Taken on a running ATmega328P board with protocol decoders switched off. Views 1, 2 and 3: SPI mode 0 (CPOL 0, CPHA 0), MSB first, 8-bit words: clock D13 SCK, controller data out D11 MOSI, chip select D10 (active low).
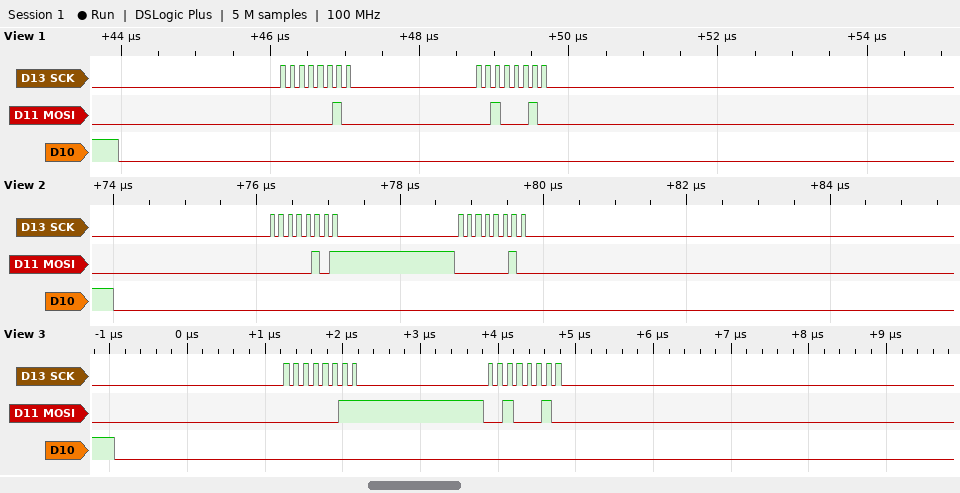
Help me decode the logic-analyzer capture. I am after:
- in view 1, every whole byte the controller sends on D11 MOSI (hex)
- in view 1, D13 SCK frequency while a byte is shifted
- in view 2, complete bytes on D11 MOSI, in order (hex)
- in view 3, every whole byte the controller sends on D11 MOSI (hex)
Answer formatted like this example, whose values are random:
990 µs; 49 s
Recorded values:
02 22; 8 MHz; 05 02; 03 22
